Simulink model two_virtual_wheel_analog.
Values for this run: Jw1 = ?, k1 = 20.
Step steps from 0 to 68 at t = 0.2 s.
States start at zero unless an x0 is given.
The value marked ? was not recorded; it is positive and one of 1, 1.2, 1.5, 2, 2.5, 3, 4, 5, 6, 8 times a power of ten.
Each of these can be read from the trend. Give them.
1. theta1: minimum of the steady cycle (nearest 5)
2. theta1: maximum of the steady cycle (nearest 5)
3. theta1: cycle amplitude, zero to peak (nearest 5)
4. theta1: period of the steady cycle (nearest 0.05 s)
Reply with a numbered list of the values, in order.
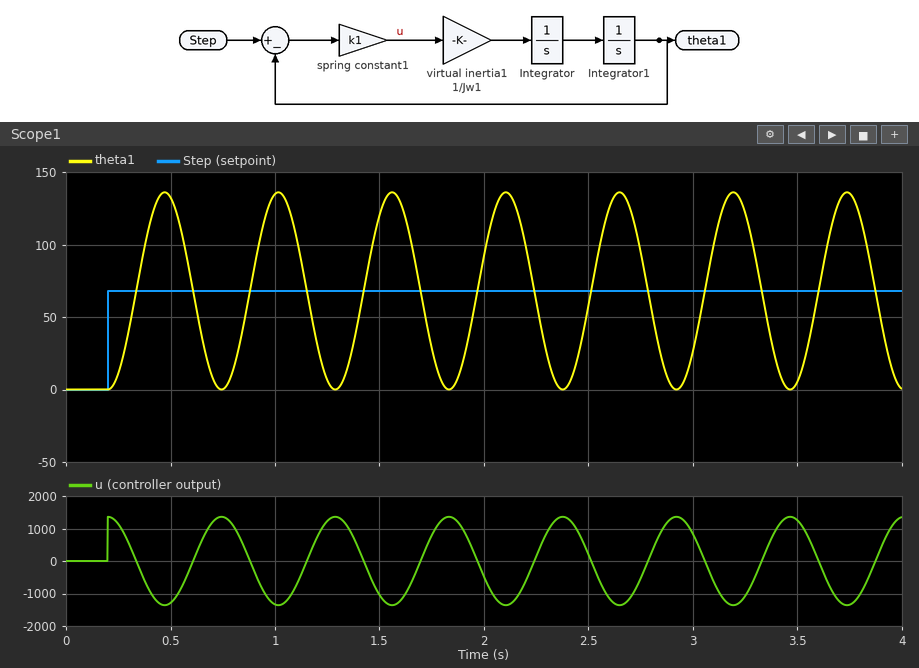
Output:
1. 0
2. 135
3. 70
4. 0.55 s
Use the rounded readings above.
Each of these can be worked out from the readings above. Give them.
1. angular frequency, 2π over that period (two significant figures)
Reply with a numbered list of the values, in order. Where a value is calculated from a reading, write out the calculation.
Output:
1. 2π / 0.55 = 11 rad/s
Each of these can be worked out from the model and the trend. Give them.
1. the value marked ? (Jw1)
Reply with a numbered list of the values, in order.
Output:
1. 0.15
